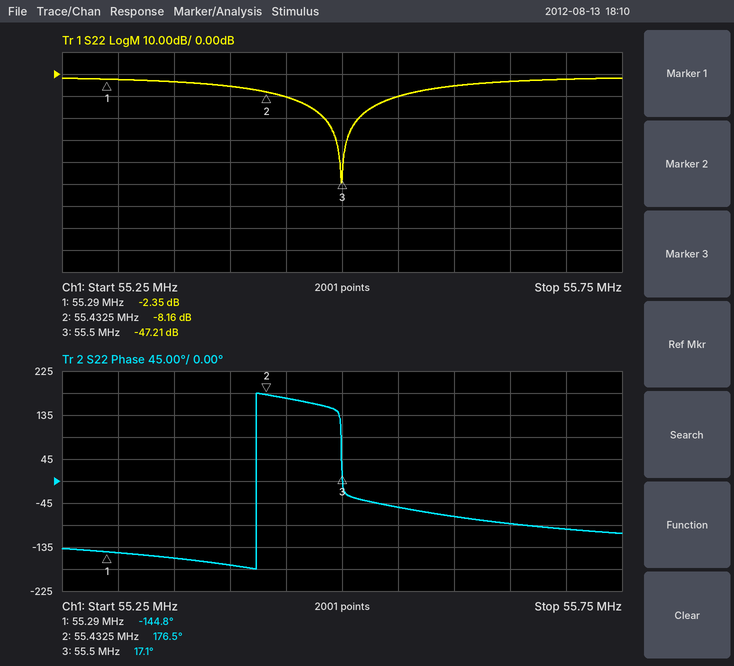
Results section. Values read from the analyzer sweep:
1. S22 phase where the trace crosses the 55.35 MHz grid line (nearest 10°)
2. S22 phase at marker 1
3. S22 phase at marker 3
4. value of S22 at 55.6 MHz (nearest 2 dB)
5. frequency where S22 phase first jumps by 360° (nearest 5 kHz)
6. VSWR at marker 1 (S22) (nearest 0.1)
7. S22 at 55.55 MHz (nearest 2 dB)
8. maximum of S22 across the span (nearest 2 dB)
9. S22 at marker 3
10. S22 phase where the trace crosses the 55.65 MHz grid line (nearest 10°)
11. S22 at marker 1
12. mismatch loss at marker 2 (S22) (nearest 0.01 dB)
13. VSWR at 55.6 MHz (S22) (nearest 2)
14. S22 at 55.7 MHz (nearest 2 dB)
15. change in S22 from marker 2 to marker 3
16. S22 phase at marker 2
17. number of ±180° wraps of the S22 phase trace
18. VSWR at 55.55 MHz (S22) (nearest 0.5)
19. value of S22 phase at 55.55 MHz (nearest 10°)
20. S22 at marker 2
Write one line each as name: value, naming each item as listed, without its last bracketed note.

S22 phase where the trace crosses the 55.35 MHz grid line: -160°
S22 phase at marker 1: -144.8°
S22 phase at marker 3: 17.1°
value of S22 at 55.6 MHz: -6 dB
frequency where S22 phase first jumps by 360°: 55.425 MHz
VSWR at marker 1 (S22): 7.4
S22 at 55.55 MHz: -10 dB
maximum of S22 across the span: -2 dB
S22 at marker 3: -47.21 dB
S22 phase where the trace crosses the 55.65 MHz grid line: -90°
S22 at marker 1: -2.35 dB
mismatch loss at marker 2 (S22): 0.72 dB
VSWR at 55.6 MHz (S22): 4
S22 at 55.7 MHz: -2 dB
change in S22 from marker 2 to marker 3: -39.05 dB
S22 phase at marker 2: 176.5°
number of ±180° wraps of the S22 phase trace: 1
VSWR at 55.55 MHz (S22): 2.0
value of S22 phase at 55.55 MHz: -50°
S22 at marker 2: -8.16 dB
